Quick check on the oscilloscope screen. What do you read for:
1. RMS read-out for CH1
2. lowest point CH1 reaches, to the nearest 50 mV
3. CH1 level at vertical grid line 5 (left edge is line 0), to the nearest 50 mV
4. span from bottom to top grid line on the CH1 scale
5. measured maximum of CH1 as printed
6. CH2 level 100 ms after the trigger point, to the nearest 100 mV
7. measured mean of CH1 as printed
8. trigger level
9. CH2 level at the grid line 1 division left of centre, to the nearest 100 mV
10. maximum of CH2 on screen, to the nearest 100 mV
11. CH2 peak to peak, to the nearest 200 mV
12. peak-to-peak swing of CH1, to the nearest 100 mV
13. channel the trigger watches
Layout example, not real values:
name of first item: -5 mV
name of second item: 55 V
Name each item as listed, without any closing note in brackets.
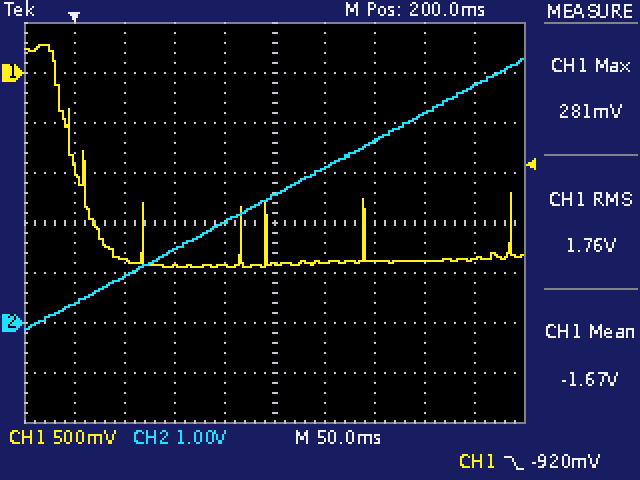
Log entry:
RMS read-out for CH1: 1.76 V
lowest point CH1 reaches, to the nearest 50 mV: -1.95 V
CH1 level at vertical grid line 5 (left edge is line 0), to the nearest 50 mV: -1.90 V
span from bottom to top grid line on the CH1 scale: 4 V
measured maximum of CH1 as printed: 281 mV
CH2 level 100 ms after the trigger point, to the nearest 100 mV: 1.5 V
measured mean of CH1 as printed: -1.67 V
trigger level: -920 mV
CH2 level at the grid line 1 division left of centre, to the nearest 100 mV: 2.0 V
maximum of CH2 on screen, to the nearest 100 mV: 5.3 V
CH2 peak to peak, to the nearest 200 mV: 5.4 V
peak-to-peak swing of CH1, to the nearest 100 mV: 2.20 V
channel the trigger watches: CH1
